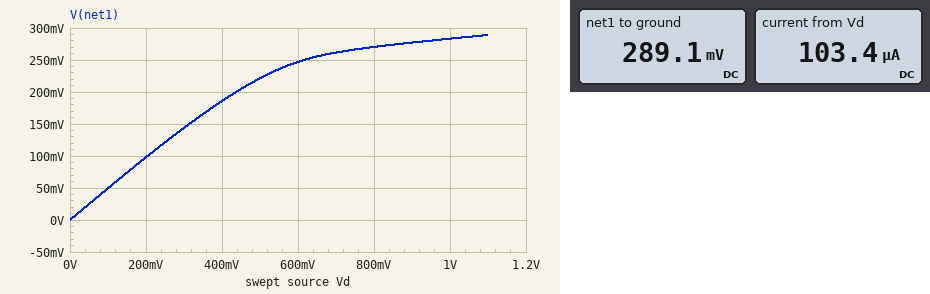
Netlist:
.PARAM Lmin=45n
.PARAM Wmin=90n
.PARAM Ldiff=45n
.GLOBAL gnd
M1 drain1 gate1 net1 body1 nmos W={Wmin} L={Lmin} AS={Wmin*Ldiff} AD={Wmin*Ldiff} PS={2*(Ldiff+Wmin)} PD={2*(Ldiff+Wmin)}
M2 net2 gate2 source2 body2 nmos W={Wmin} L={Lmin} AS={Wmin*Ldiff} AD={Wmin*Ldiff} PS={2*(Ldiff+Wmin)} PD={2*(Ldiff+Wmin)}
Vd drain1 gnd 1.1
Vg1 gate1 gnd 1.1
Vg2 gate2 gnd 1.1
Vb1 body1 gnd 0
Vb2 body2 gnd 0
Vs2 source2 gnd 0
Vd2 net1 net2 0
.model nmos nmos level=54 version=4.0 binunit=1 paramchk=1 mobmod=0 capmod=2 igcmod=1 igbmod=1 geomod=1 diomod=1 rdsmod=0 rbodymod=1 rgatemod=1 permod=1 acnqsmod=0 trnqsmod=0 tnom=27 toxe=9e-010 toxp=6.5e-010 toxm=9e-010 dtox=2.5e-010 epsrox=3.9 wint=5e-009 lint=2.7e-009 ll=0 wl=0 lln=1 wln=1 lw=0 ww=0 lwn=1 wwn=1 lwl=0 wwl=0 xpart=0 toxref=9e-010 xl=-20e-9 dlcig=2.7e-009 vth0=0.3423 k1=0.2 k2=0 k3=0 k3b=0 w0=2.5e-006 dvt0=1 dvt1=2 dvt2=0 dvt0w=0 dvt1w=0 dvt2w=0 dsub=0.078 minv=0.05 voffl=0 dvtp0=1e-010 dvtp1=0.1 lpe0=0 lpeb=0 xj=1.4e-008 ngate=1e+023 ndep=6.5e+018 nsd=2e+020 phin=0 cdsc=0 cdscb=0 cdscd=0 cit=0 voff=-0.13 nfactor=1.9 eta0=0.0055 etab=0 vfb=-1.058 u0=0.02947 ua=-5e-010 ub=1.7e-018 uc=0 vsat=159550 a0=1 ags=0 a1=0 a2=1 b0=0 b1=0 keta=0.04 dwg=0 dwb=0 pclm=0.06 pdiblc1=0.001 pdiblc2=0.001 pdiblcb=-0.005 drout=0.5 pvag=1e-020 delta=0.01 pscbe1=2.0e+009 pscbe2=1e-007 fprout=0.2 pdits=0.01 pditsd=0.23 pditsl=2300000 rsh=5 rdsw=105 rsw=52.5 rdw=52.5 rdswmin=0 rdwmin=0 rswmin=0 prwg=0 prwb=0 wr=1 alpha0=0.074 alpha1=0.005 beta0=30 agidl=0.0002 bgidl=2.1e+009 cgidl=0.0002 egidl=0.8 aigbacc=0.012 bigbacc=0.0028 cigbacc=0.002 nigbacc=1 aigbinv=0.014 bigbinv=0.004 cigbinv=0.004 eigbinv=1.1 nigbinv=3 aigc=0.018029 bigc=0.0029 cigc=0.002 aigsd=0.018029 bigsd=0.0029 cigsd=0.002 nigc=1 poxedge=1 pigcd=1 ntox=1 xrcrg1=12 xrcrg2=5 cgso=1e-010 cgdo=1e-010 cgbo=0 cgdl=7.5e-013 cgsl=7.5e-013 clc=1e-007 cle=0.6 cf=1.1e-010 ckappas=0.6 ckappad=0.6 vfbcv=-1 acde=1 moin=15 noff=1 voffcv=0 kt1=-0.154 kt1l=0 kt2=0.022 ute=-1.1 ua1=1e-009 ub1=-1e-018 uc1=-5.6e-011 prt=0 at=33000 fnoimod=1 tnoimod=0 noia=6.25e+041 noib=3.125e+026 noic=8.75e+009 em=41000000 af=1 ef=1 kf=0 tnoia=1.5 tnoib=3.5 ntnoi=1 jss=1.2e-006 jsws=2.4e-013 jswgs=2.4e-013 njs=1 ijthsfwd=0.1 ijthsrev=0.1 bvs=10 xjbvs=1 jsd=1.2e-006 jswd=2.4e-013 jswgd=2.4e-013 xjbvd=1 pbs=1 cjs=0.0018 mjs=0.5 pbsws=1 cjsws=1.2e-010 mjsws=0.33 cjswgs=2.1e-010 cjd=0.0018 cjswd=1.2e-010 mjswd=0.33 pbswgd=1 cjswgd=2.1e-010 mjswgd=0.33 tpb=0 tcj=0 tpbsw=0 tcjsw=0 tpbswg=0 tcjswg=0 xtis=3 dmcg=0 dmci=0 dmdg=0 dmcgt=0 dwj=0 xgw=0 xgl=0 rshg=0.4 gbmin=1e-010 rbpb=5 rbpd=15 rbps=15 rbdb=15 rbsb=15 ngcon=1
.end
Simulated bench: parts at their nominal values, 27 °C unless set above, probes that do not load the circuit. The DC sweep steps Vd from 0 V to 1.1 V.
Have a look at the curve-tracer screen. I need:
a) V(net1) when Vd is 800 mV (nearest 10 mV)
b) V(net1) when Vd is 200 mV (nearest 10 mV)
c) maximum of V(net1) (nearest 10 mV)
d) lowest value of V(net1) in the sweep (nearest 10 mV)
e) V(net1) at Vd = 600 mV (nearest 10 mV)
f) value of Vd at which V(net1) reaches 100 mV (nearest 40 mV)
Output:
270 mV
100 mV
290 mV
0 V
250 mV
200 mV
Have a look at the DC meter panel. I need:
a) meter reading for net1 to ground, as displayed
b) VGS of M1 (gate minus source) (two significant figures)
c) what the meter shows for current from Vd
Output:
289.1 mV
810 mV
103.4 µA
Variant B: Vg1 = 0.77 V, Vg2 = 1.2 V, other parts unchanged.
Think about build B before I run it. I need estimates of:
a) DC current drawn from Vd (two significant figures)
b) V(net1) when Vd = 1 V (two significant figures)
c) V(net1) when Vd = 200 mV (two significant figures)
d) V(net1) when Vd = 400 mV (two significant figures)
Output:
66 µA
160 mV
85 mV
130 mV
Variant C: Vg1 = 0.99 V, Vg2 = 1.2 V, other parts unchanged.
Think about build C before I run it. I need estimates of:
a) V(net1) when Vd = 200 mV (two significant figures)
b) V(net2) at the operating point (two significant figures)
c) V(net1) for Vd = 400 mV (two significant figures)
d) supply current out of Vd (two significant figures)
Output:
95 mV
240 mV
170 mV
93 µA
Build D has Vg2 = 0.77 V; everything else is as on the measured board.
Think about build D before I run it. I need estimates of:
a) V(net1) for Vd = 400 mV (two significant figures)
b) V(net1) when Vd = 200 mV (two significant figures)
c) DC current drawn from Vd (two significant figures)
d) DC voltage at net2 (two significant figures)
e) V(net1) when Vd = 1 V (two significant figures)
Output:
210 mV
110 mV
85 µA
360 mV
350 mV
